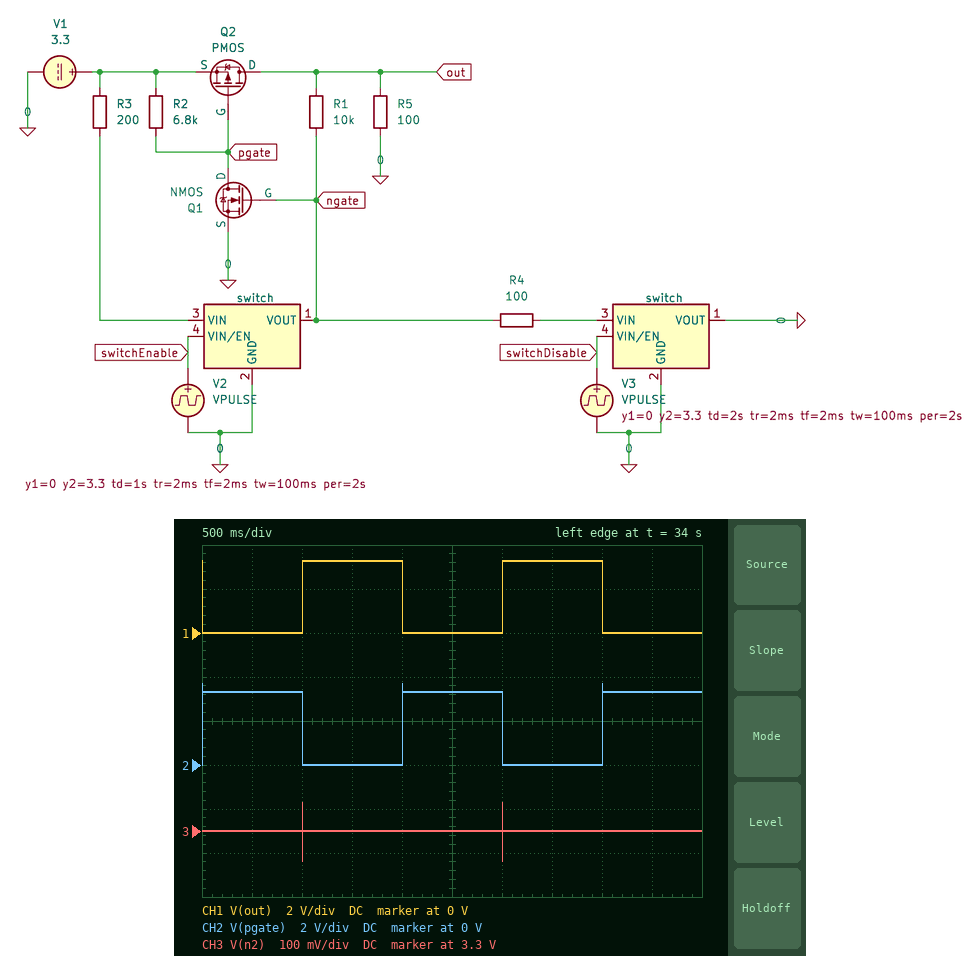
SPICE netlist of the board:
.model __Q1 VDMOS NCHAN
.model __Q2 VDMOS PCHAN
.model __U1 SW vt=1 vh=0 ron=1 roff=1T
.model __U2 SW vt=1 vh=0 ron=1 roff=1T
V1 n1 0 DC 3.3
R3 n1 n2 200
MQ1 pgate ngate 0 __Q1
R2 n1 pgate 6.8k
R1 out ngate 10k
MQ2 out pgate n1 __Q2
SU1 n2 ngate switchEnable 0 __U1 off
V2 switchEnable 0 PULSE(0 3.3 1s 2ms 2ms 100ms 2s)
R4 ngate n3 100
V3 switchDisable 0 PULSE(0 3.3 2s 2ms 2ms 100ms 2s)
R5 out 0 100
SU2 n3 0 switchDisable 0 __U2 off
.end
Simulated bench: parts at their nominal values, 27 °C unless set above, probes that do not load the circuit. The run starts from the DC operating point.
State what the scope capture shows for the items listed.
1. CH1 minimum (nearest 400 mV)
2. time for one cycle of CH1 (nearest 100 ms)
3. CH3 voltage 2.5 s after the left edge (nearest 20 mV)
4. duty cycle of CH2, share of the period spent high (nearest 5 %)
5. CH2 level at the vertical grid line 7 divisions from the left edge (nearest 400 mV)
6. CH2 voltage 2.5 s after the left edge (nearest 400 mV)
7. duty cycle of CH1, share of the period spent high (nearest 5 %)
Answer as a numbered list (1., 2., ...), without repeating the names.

1. 0 V
2. 2.0 s
3. 3.30 V
4. 50 %
5. 0 V
6. 3.2 V
7. 50 %
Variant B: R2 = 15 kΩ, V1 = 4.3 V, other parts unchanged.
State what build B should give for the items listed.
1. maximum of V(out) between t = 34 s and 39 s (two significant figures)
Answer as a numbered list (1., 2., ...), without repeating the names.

1. 4.3 V
